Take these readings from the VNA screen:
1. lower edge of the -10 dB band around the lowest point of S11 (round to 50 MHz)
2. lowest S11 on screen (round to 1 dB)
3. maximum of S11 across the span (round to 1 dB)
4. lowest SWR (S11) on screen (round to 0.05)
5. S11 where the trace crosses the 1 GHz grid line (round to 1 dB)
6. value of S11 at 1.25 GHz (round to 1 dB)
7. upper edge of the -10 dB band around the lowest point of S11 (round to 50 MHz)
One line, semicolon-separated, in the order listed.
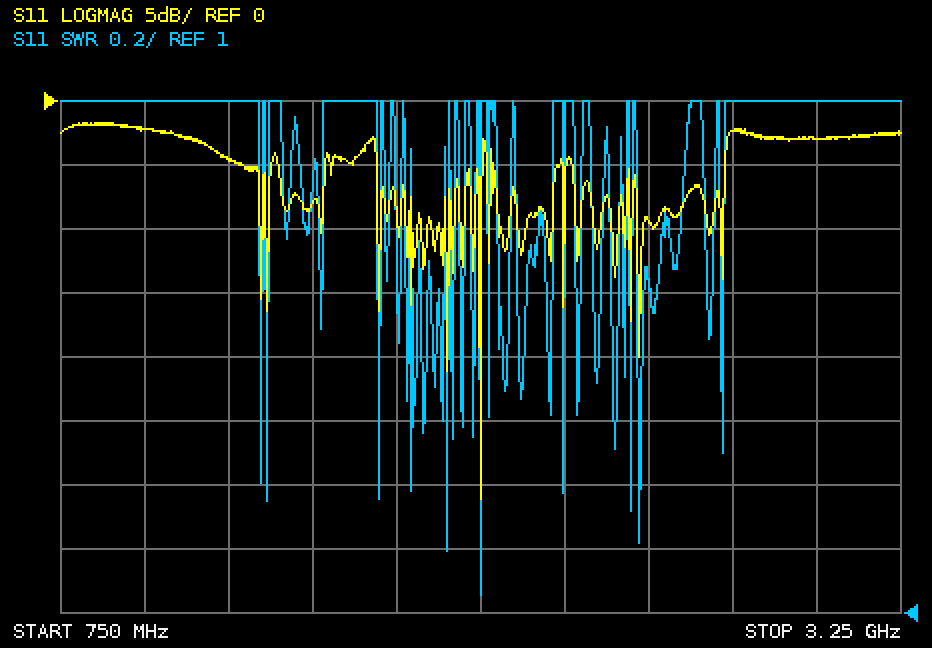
2.00 GHz; -31 dB; -2 dB; 1.05; -2 dB; -5 dB; 2.00 GHz
